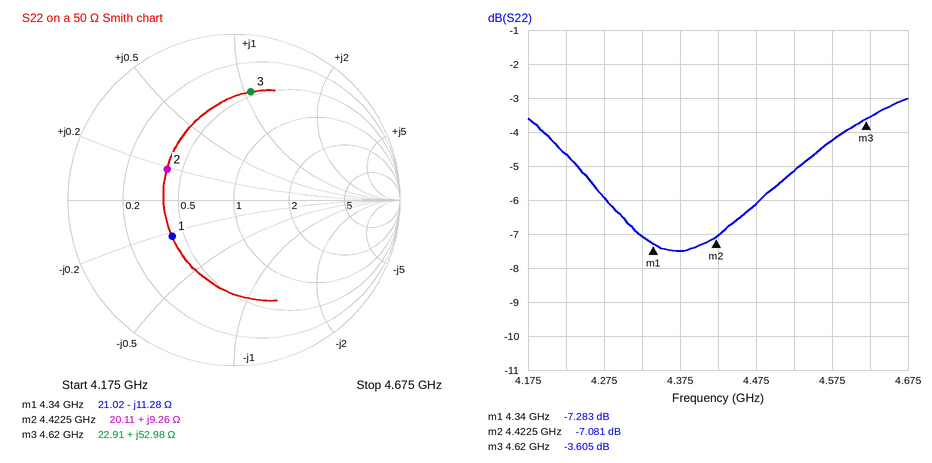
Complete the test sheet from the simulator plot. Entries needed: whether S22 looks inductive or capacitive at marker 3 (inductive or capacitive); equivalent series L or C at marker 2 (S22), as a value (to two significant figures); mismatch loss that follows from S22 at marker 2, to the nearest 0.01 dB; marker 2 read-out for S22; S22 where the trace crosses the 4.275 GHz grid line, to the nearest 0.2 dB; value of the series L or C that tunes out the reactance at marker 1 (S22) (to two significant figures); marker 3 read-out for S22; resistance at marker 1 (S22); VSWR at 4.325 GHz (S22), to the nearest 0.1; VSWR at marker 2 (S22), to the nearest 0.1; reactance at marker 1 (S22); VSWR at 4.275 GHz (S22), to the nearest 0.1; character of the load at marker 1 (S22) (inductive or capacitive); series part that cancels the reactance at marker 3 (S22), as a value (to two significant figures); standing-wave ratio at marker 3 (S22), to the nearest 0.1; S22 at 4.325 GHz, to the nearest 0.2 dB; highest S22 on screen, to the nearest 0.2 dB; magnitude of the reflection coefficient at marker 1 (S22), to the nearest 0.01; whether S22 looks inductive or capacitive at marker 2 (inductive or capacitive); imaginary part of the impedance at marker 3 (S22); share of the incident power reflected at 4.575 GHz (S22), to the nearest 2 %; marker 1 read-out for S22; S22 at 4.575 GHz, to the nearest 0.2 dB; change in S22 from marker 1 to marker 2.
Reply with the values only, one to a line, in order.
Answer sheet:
inductive
330 pH
0.95 dB
-7.081 dB
-6.0 dB
410 pH
-3.605 dB
21.02 Ω
2.6
2.6
-11.28 Ω
3.0
capacitive
650 fF
4.9
-7.0 dB
-3.0 dB
0.43
inductive
+52.98 Ω
38 %
-7.283 dB
-4.2 dB
0.202 dB
